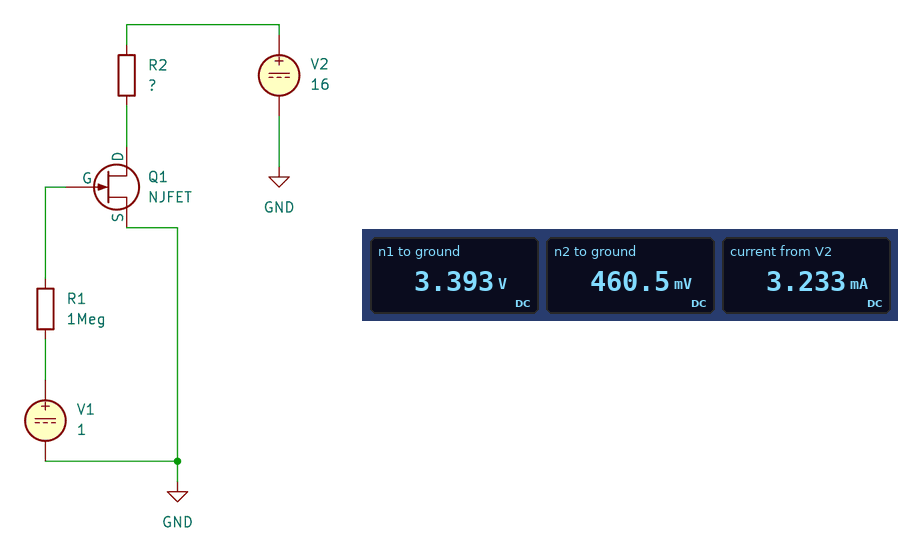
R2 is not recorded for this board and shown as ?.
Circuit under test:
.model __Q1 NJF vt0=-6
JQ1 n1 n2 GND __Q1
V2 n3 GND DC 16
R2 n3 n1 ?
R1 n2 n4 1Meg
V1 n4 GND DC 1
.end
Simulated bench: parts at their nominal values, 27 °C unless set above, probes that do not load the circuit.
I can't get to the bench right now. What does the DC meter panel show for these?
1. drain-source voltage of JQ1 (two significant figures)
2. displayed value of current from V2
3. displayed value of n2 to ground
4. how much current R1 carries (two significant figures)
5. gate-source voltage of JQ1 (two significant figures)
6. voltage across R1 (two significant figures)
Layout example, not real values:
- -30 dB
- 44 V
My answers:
- 3.4 V
- 3.233 mA
- 460.5 mV
- 540 nA
- 460 mV
- 540 mV
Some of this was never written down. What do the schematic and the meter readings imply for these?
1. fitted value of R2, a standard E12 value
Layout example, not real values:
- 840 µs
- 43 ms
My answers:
- 3.9 kΩ
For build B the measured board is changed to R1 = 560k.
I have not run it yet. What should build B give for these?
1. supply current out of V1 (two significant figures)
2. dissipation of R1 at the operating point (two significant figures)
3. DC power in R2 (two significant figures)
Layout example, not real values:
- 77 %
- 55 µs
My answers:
- 940 nA
- 490 nW
- 41 mW
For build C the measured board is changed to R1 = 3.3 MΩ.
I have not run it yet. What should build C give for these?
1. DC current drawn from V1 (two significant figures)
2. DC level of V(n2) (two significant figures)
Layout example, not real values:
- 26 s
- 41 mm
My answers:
- 170 nA
- 430 mV
